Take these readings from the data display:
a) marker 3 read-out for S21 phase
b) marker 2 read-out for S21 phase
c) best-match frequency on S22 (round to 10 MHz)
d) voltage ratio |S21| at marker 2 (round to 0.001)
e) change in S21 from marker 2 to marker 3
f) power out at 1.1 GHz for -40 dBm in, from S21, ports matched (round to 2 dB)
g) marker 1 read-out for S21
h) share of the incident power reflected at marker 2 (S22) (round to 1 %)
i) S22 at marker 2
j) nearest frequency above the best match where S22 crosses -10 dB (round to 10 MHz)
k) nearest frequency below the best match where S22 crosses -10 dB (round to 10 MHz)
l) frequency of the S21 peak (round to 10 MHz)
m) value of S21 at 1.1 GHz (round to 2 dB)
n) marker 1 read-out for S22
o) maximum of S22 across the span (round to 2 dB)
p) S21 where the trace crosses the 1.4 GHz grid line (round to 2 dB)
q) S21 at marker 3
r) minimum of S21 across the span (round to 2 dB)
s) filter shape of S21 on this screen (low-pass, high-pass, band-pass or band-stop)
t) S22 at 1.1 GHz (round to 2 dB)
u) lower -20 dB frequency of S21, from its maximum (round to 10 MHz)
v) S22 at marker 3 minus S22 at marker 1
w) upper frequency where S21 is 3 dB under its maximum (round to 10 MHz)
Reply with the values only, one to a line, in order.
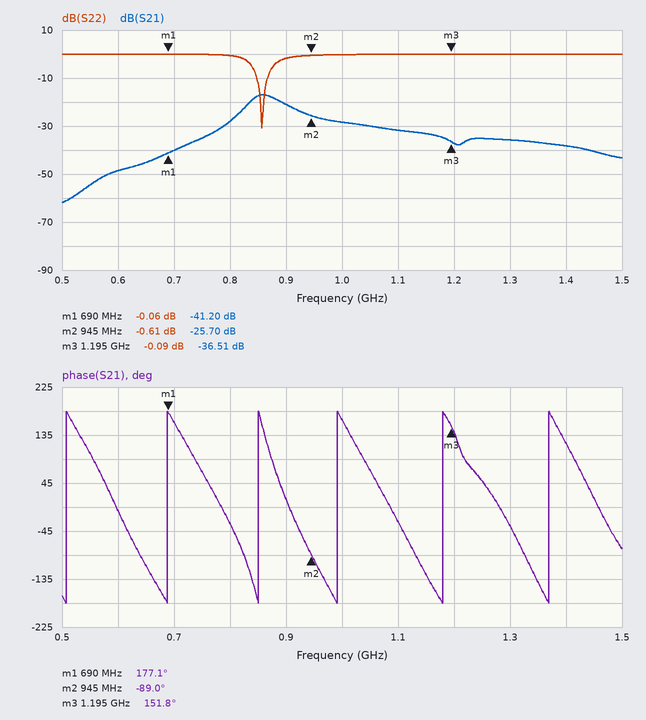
151.8°
-89.0°
860 MHz
0.052
-10.81 dB
-72 dBm
-41.20 dB
87 %
-0.61 dB
870 MHz
850 MHz
860 MHz
-32 dB
-0.06 dB
0 dB
-38 dB
-36.51 dB
-62 dB
band-pass
0 dB
730 MHz
-0.03 dB
890 MHz
